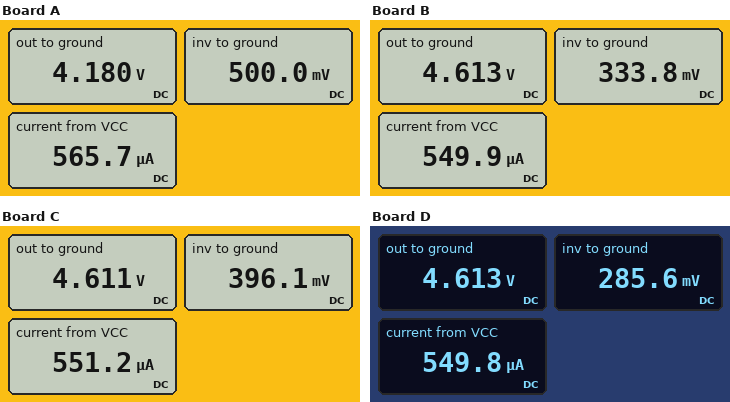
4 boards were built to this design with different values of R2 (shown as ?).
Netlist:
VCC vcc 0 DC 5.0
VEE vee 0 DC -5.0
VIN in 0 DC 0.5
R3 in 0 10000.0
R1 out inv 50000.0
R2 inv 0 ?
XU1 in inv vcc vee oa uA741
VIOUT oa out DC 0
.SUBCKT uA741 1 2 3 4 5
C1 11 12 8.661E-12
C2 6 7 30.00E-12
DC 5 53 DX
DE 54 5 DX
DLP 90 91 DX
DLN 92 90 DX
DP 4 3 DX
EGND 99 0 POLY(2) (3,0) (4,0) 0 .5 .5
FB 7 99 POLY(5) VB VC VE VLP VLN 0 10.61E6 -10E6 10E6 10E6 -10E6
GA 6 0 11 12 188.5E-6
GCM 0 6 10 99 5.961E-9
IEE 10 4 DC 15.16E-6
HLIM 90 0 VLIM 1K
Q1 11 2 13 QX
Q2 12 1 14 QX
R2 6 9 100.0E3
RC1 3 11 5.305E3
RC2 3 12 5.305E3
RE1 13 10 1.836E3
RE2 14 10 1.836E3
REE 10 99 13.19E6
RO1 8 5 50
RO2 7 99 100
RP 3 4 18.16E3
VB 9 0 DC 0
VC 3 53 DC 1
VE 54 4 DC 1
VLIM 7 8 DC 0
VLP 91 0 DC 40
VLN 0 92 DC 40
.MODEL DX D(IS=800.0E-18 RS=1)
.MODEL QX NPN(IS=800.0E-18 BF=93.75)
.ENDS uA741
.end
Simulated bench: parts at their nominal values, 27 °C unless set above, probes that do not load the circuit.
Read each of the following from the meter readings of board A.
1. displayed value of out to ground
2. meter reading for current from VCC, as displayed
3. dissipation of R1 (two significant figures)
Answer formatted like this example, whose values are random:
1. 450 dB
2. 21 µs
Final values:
1. 4.180 V
2. 565.7 µA
3. 270 µW
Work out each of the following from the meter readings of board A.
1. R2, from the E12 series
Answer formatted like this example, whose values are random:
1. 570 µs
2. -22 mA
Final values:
1. 6.8 kΩ
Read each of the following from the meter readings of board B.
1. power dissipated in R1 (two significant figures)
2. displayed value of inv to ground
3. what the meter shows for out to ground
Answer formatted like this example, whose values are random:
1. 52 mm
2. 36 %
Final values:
1. 370 µW
2. 333.8 mV
3. 4.613 V
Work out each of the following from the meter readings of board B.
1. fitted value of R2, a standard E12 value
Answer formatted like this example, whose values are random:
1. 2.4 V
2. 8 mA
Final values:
1. 3.9 kΩ
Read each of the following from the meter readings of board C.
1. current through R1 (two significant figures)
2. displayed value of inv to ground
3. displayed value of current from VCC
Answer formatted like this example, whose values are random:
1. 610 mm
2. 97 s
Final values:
1. 84 µA
2. 396.1 mV
3. 551.2 µA
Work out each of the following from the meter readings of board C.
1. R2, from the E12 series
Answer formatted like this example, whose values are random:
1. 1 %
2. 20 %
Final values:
1. 4.7 kΩ
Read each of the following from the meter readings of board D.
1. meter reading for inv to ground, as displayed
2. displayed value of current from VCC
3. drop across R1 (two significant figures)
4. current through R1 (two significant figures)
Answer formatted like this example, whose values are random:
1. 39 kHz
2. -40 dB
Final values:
1. 285.6 mV
2. 549.8 µA
3. 4.3 V
4. 87 µA
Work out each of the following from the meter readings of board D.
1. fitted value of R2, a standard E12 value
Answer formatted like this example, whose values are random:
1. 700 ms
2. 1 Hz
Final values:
1. 3.3 kΩ
